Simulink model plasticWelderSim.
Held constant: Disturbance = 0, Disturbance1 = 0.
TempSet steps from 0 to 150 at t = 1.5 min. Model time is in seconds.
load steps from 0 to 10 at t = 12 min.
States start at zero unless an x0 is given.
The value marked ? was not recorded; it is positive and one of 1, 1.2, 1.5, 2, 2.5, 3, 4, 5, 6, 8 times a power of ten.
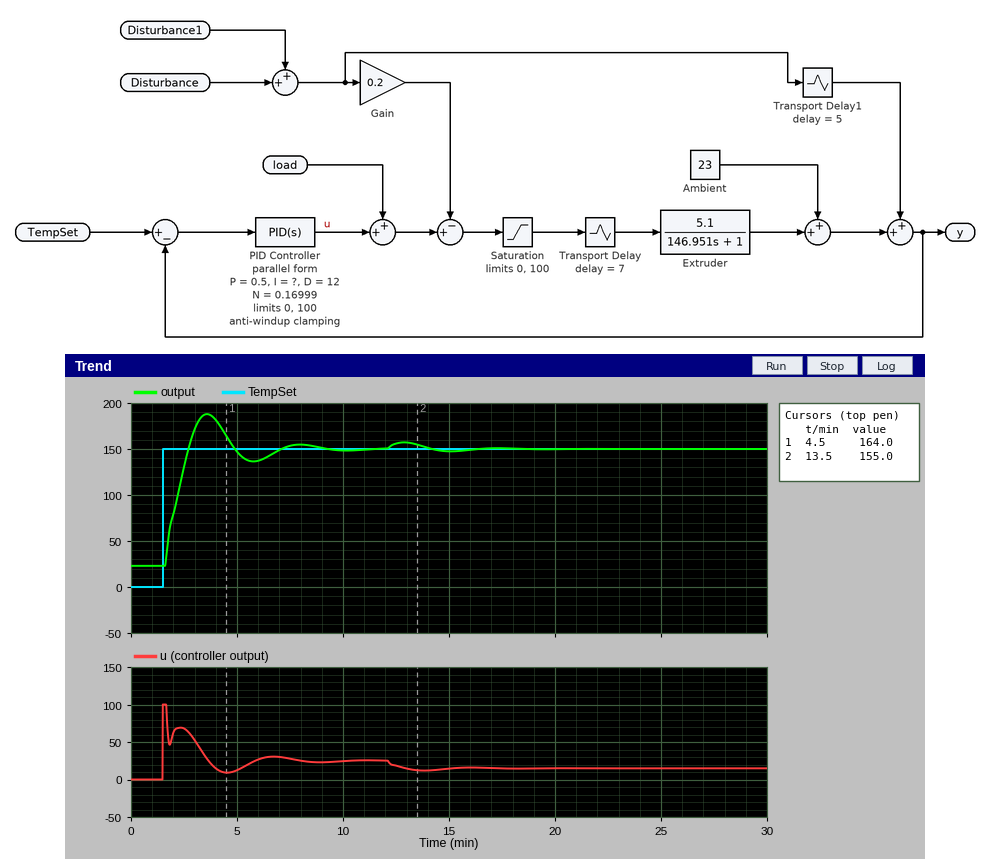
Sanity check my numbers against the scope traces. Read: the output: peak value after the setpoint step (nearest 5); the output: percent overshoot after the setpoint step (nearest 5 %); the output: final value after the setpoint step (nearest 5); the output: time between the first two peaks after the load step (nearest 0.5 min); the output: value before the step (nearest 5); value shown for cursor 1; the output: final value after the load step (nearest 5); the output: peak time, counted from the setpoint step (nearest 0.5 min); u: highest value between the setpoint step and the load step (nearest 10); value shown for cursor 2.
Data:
190
30 %
150
4.5 min
25
164.0
150
2.0 min
100
155.0
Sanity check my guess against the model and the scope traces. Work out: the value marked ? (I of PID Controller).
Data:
0.025
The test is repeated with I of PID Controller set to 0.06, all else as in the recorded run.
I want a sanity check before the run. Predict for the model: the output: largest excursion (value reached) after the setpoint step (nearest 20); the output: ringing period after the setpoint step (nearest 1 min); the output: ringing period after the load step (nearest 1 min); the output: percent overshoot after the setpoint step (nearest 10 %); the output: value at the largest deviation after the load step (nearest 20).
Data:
200
3 min
3 min
40 %
160
